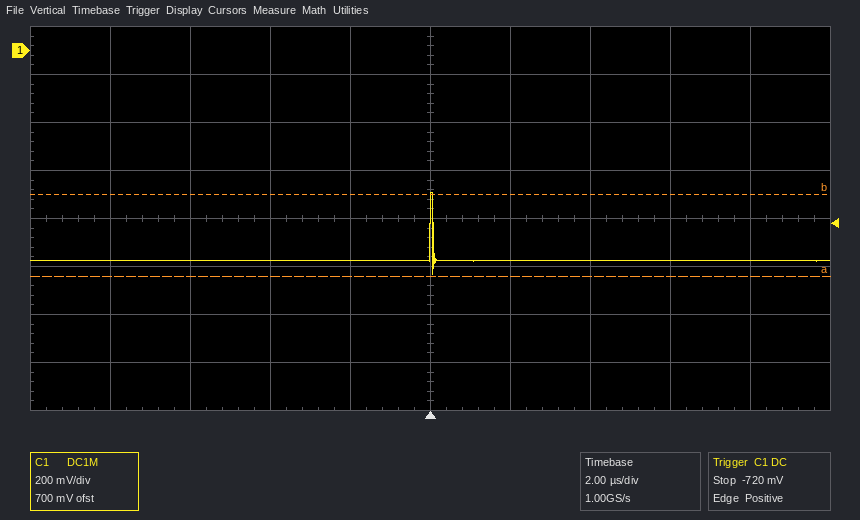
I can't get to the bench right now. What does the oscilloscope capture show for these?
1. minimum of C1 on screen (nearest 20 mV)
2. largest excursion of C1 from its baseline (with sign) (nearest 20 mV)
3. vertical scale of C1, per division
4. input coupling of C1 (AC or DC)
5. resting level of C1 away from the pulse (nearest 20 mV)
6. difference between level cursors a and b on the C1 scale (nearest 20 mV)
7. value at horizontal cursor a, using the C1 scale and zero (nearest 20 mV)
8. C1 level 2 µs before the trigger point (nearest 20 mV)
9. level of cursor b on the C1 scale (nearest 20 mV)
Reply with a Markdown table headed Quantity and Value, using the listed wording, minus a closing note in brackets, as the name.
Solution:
| Quantity | Value |
|---|---|
| minimum of C1 on screen | -940 mV |
| largest excursion of C1 from its baseline (with sign) | +280 mV |
| vertical scale of C1, per division | 200 mV |
| input coupling of C1 | DC |
| resting level of C1 away from the pulse | -880 mV |
| difference between level cursors a and b on the C1 scale | 340 mV |
| value at horizontal cursor a, using the C1 scale and zero | -940 mV |
| C1 level 2 µs before the trigger point | -880 mV |
| level of cursor b on the C1 scale | -600 mV |
